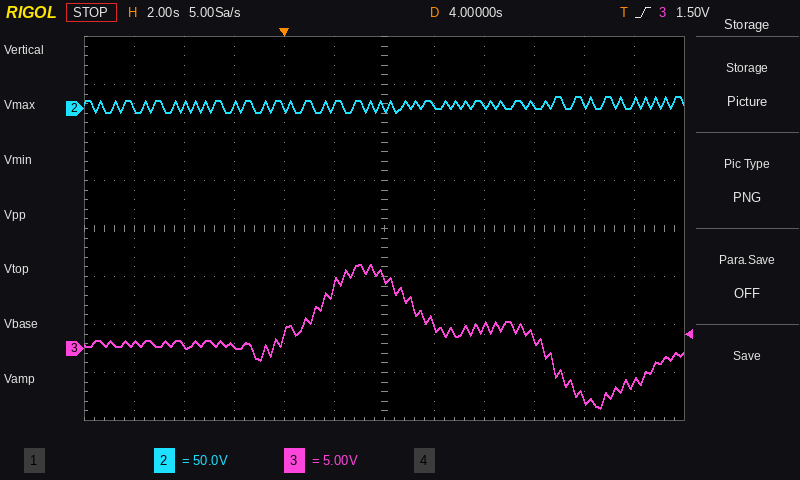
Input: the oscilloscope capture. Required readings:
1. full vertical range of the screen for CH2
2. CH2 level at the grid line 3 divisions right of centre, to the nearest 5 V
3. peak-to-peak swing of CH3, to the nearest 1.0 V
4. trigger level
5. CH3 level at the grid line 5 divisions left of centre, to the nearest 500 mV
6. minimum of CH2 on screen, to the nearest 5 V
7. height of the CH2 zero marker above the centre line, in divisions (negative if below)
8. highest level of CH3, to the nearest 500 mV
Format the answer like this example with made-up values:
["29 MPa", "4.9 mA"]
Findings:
["400 V", "5 V", "15.0 V", "1.50 V", "500 mV", "-5 V", "+2.5 div", "9.0 V"]
